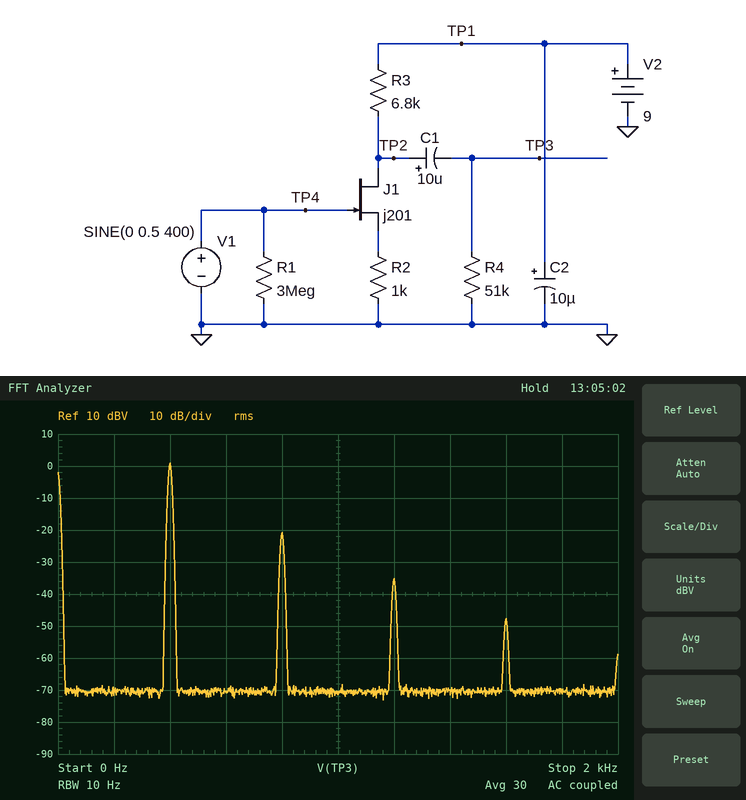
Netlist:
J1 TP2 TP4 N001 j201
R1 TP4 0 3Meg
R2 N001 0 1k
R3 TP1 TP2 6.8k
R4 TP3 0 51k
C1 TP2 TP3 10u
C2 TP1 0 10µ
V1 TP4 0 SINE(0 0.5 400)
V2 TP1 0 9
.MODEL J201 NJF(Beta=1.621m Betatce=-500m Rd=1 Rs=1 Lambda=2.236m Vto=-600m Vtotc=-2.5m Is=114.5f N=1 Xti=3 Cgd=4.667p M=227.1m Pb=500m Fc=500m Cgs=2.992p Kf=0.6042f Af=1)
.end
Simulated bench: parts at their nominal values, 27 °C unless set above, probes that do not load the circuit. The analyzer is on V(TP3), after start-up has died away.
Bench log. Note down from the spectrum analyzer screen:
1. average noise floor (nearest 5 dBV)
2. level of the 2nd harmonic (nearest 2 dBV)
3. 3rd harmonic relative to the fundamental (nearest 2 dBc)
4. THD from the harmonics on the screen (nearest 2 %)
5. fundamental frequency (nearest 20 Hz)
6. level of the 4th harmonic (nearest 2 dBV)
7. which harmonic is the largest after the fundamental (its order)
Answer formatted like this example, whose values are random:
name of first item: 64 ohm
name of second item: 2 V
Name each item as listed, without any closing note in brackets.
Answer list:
average noise floor: -70 dBV
level of the 2nd harmonic: -20 dBV
3rd harmonic relative to the fundamental: -36 dBc
THD from the harmonics on the screen: 8 %
fundamental frequency: 400 Hz
level of the 4th harmonic: -48 dBV
which harmonic is the largest after the fundamental: 2
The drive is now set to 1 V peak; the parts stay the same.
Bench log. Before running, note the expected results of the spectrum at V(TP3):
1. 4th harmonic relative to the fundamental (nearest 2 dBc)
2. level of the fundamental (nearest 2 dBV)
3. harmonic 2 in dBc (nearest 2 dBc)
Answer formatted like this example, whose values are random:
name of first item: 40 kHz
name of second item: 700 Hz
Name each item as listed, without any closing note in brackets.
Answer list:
4th harmonic relative to the fundamental: -58 dBc
level of the fundamental: 6 dBV
harmonic 2 in dBc: -12 dBc
